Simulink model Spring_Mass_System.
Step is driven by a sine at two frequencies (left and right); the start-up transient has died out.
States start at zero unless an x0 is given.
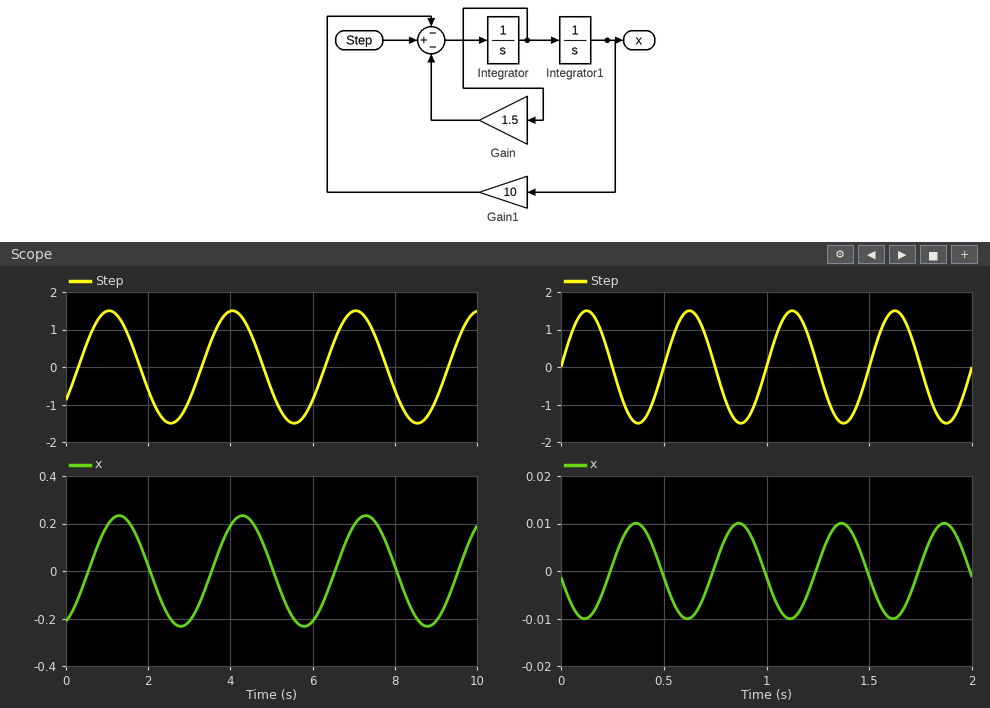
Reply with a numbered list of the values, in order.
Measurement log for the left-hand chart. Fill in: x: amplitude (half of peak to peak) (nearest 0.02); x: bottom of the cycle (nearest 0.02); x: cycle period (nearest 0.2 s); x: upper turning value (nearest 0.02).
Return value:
1. 0.24
2. -0.24
3. 3.0 s
4. 0.24
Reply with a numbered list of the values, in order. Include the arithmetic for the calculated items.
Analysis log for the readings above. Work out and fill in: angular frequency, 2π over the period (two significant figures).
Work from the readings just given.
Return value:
1. 2π / 3 = 2.1 rad/s
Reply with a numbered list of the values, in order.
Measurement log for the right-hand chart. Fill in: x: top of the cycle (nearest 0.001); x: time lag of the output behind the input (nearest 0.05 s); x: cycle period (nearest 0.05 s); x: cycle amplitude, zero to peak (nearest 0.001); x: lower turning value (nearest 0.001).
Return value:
1. 0.010
2. 0.25 s
3. 0.50 s
4. 0.010
5. -0.010
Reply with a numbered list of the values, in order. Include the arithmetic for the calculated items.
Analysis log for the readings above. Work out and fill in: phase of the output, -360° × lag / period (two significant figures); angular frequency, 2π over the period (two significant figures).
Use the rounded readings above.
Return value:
1. -360 × 0.25 / 0.5 = -180°
2. 2π / 0.5 = 13 rad/s
